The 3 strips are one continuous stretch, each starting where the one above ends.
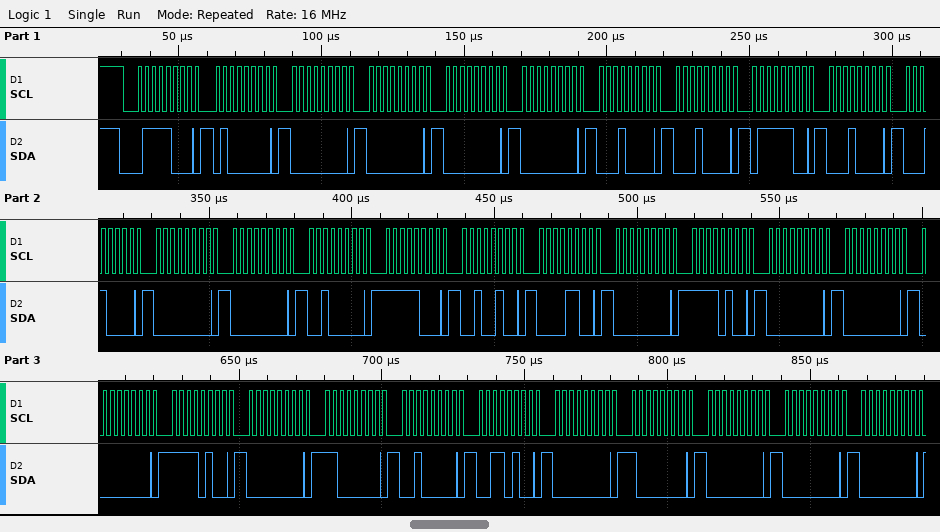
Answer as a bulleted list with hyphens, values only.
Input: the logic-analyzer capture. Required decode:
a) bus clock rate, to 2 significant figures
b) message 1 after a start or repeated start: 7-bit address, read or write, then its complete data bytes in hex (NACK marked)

- 400 kHz
- 0x3C write: 40 00 00 00 00 10 10 7C 10 10 00 00 20 F8 24 0C 00 F4 00 00 00 F4 00 C0 20 34 00 80 00 00 00
